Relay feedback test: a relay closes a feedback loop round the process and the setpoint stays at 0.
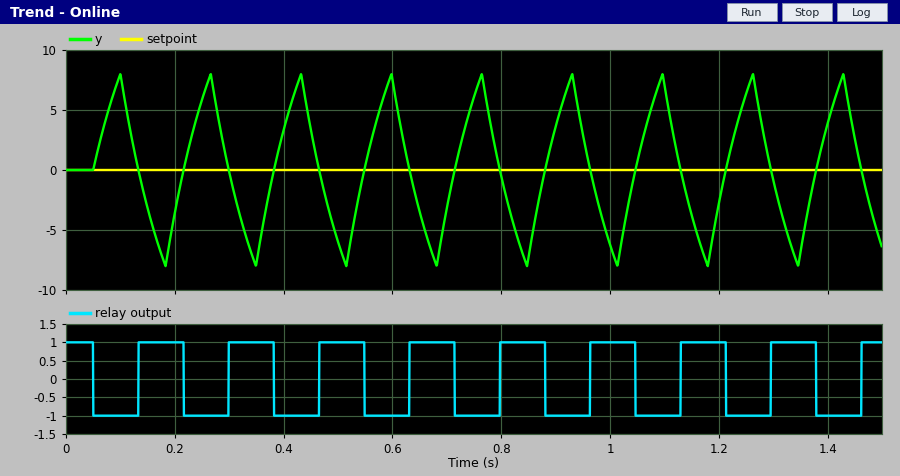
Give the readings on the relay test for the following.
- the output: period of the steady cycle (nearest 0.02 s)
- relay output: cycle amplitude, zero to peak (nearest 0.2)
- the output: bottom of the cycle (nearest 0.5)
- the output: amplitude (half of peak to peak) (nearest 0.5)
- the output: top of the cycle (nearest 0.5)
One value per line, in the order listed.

0.16 s
1.0
-8.0
8.0
8.0
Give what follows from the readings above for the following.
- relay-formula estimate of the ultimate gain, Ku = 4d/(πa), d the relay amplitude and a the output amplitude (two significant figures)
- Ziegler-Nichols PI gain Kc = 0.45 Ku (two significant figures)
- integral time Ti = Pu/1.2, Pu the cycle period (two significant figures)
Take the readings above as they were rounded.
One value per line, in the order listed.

0.16
0.072
0.13 s
